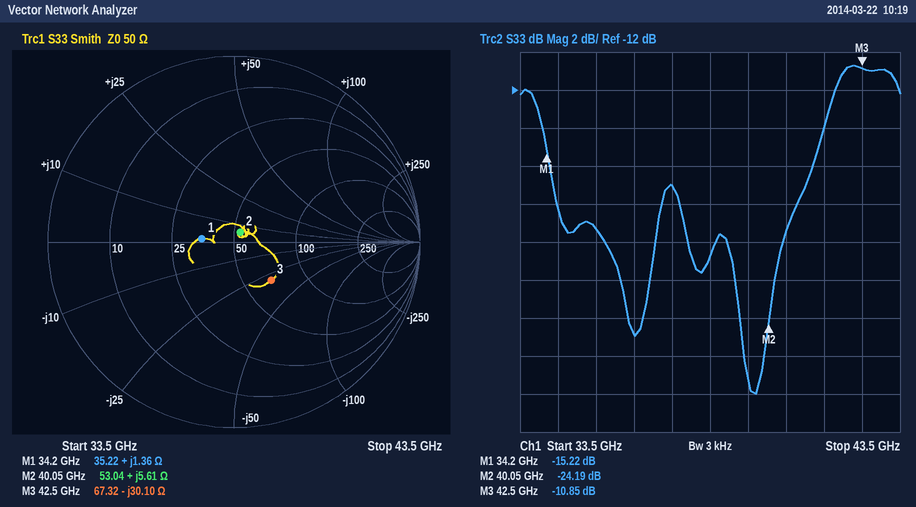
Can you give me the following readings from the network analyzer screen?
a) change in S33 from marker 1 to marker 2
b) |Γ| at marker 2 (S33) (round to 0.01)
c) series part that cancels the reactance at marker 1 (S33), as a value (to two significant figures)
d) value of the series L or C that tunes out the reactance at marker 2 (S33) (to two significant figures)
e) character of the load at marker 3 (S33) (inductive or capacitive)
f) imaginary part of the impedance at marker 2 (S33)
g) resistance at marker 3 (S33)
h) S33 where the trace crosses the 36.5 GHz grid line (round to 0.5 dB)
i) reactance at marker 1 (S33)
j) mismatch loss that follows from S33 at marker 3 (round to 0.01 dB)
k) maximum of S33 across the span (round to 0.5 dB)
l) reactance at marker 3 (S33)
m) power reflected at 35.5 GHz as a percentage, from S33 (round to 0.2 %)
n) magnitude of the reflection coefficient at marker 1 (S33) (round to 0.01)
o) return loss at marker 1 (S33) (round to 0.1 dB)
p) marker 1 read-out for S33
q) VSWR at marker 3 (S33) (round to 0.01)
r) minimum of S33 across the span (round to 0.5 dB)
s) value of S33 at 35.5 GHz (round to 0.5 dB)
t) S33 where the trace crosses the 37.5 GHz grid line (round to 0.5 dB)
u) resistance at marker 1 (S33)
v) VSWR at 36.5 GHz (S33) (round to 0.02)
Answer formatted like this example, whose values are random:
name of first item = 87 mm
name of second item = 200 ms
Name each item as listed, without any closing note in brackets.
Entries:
change in S33 from marker 1 to marker 2 = -8.97 dB
|Γ| at marker 2 (S33) = 0.06
series part that cancels the reactance at marker 1 (S33), as a value = 3.4 pF
value of the series L or C that tunes out the reactance at marker 2 (S33) = 710 fF
character of the load at marker 3 (S33) = capacitive
imaginary part of the impedance at marker 2 = +5.61 Ω
resistance at marker 3 = 67.32 Ω
S33 where the trace crosses the 36.5 GHz grid line = -25.0 dB
reactance at marker 1 = +1.36 Ω
mismatch loss that follows from S33 at marker 3 = 0.37 dB
maximum of S33 across the span = -10.5 dB
reactance at marker 3 = -30.10 Ω
power reflected at 35.5 GHz as a percentage, from S33 = 1.2 %
magnitude of the reflection coefficient at marker 1 (S33) = 0.17
return loss at marker 1 (S33) = 15.2 dB
marker 1 read-out for S33 = -15.22 dB
VSWR at marker 3 (S33) = 1.80
minimum of S33 across the span = -28.0 dB
value of S33 at 35.5 GHz = -19.5 dB
S33 where the trace crosses the 37.5 GHz grid line = -17.0 dB
resistance at marker 1 = 35.22 Ω
VSWR at 36.5 GHz (S33) = 1.12
